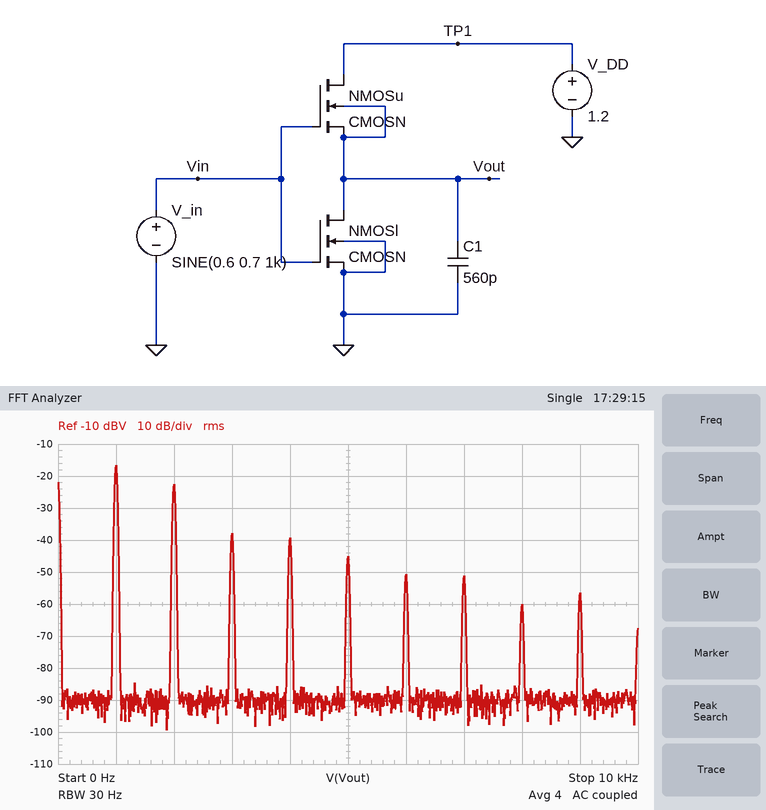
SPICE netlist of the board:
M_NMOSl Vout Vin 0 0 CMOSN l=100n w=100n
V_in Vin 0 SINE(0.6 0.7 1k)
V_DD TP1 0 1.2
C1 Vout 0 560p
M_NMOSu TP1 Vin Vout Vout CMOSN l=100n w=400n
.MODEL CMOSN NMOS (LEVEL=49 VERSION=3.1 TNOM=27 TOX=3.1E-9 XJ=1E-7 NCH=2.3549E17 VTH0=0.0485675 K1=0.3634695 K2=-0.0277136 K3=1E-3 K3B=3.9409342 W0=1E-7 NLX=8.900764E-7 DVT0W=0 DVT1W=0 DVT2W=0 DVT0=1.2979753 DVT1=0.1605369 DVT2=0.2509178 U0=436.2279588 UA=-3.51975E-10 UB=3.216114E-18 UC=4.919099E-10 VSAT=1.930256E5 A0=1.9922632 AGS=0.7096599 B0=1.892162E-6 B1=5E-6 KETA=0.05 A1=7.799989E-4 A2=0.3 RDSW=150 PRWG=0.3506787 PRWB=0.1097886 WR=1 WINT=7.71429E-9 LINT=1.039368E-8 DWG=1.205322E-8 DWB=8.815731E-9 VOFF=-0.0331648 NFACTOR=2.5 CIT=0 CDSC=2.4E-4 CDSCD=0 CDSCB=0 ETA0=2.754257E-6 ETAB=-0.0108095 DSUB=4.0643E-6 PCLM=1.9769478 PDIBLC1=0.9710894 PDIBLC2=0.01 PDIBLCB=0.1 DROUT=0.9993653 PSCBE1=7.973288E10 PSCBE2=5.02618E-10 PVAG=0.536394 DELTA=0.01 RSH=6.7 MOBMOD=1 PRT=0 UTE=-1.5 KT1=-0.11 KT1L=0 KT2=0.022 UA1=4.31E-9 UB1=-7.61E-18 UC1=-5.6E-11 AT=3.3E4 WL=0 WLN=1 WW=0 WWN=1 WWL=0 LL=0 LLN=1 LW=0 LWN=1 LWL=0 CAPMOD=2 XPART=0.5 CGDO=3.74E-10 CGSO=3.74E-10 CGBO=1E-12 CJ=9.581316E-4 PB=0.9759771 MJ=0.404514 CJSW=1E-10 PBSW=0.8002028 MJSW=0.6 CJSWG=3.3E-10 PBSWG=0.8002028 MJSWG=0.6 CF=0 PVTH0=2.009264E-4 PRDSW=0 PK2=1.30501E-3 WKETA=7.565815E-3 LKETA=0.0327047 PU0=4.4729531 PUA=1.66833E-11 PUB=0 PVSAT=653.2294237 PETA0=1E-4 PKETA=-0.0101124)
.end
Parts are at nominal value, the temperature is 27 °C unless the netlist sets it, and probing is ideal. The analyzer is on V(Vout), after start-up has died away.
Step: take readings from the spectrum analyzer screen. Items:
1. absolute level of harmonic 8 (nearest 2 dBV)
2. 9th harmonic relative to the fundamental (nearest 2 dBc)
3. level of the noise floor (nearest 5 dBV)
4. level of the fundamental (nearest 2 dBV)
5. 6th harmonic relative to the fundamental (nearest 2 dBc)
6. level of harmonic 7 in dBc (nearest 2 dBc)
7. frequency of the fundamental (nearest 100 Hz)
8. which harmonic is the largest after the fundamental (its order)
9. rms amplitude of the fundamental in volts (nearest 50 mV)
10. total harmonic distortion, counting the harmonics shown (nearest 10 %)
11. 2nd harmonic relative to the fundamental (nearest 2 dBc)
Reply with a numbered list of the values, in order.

1. -60 dBV
2. -40 dBc
3. -90 dBV
4. -16 dBV
5. -34 dBc
6. -34 dBc
7. 1.0 kHz
8. 2
9. 150 mV
10. 50 %
11. -6 dBc
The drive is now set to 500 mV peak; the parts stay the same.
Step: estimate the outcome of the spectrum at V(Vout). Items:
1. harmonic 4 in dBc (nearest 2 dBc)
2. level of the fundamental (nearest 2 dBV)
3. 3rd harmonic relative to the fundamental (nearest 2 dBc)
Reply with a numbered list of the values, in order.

1. -24 dBc
2. -20 dBV
3. -20 dBc
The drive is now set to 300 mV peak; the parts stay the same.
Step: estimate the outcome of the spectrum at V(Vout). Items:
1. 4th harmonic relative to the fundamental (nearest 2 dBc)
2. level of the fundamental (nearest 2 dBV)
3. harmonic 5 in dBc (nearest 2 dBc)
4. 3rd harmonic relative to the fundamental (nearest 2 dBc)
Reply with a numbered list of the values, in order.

1. -28 dBc
2. -26 dBV
3. -30 dBc
4. -18 dBc
